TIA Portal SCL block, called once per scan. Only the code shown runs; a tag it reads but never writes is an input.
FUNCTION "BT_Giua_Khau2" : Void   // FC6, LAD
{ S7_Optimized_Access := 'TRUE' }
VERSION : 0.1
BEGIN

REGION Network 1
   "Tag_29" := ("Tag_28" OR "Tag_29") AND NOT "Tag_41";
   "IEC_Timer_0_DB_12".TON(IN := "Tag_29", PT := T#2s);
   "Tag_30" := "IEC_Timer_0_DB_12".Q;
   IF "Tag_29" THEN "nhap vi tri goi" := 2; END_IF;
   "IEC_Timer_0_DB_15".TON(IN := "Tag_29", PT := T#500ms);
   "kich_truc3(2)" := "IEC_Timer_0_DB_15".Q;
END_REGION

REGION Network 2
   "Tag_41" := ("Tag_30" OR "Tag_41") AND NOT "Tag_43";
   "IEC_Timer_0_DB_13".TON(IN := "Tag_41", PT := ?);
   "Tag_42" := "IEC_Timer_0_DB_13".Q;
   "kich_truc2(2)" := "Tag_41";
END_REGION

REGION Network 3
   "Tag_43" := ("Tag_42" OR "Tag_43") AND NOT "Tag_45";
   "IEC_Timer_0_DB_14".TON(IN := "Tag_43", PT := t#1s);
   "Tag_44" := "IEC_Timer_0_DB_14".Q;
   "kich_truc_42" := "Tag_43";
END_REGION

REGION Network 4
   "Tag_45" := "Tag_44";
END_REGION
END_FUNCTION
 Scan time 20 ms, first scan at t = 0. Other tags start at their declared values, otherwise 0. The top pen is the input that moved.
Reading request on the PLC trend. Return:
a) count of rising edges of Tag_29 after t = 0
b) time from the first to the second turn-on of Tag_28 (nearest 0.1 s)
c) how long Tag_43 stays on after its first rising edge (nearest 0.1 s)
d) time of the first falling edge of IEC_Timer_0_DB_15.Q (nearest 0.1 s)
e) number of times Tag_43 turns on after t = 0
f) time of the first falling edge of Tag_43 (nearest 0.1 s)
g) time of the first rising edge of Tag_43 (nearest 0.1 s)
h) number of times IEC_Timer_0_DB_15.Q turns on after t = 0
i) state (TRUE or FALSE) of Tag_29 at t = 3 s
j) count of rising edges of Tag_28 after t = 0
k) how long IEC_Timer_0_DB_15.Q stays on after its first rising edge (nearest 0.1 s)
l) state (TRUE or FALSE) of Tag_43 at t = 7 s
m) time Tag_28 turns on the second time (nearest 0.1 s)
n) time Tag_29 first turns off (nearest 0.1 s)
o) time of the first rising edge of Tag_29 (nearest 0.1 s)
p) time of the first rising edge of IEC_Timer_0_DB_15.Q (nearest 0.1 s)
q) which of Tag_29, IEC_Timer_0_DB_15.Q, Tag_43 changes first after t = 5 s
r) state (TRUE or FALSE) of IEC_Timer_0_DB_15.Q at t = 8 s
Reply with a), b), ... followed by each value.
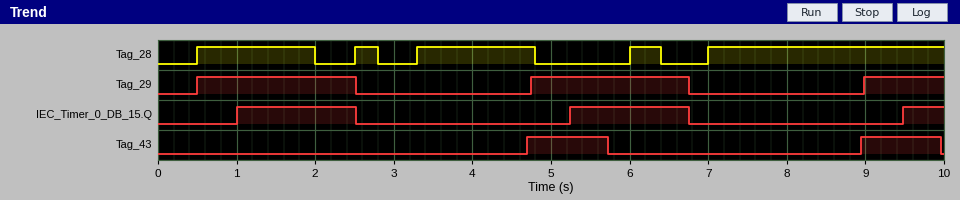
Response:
a) 3
b) 2.0 s
c) 1.0 s
d) 2.5 s
e) 2
f) 5.7 s
g) 4.7 s
h) 3
i) FALSE
j) 5
k) 1.5 s
l) FALSE
m) 2.5 s
n) 2.5 s
o) 0.5 s
p) 1.0 s
q) IEC_Timer_0_DB_15.Q
r) FALSE
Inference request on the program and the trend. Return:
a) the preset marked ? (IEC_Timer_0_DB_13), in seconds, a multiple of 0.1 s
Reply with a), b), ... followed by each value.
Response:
a) 2.2 s
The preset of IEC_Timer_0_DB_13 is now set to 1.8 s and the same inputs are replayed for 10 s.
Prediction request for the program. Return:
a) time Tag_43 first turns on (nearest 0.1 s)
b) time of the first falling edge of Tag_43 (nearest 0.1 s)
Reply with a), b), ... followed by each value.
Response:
a) 4.3 s
b) 5.3 s
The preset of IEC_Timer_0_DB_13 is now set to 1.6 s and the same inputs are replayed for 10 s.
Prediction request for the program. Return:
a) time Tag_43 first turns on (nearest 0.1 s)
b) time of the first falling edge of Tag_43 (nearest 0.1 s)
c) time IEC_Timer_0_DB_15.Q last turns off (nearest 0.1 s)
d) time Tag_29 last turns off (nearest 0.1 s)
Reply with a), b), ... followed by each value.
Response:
a) 4.1 s
b) 5.1 s
c) 9.8 s
d) 9.8 s
